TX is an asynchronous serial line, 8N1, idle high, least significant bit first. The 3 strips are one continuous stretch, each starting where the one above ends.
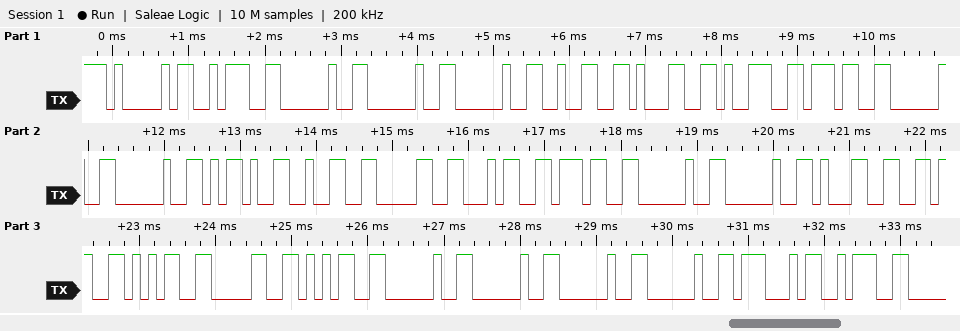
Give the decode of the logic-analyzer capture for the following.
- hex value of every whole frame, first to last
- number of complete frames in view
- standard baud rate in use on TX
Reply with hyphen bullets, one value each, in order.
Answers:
- 41 3A 20 20 20 32 31 39 37 20 20 2D 32 30 34 37 20 20 31 36 35 30 35 20 20 20 20 47 3A
- 29
- 9600 baud
